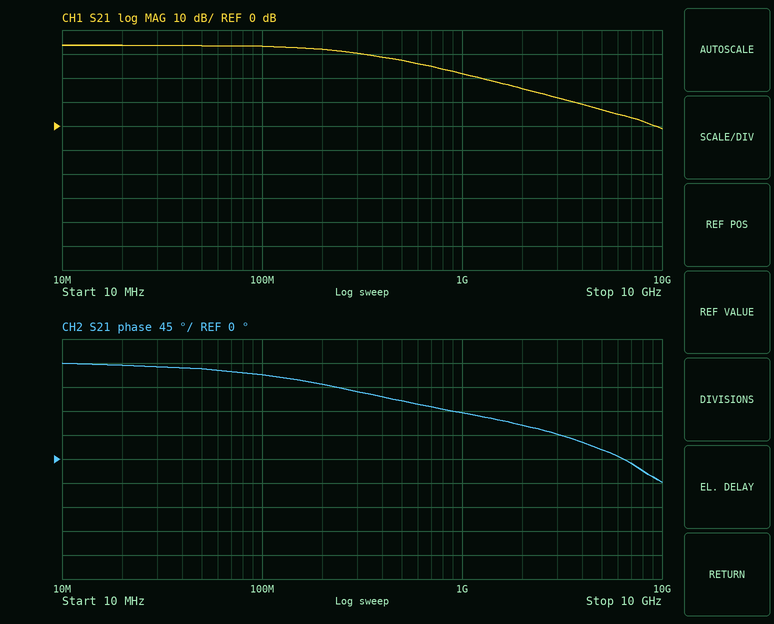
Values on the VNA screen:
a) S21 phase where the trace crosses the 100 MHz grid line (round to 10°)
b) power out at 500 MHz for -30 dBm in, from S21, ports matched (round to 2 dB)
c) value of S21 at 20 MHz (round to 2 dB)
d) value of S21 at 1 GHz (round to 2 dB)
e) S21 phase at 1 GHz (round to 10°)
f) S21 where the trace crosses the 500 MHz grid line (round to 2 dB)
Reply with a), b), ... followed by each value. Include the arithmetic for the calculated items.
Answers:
a) 160°
b) -30 dBm + (28 dB) = -2 dBm
c) 34 dB
d) 22 dB
e) 90°
f) 28 dB
